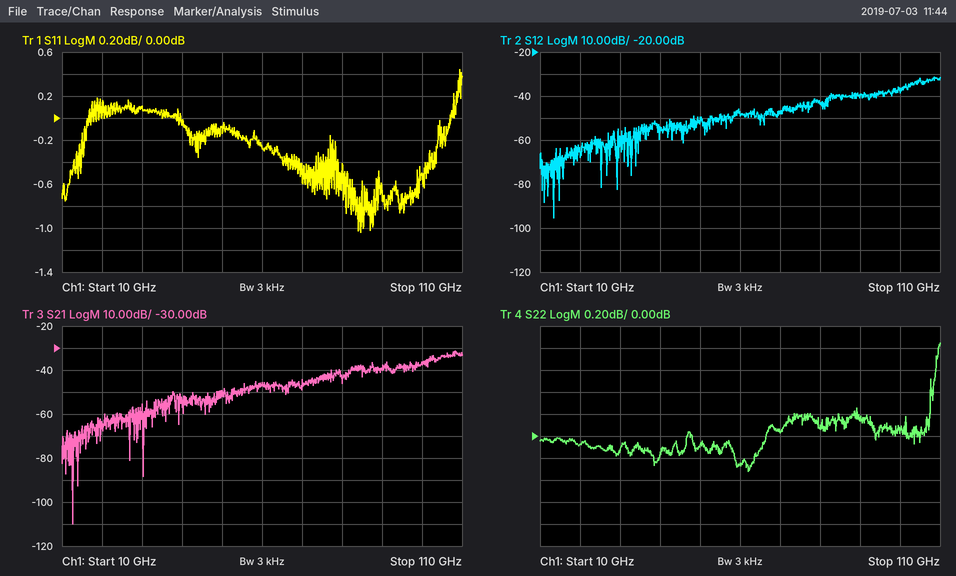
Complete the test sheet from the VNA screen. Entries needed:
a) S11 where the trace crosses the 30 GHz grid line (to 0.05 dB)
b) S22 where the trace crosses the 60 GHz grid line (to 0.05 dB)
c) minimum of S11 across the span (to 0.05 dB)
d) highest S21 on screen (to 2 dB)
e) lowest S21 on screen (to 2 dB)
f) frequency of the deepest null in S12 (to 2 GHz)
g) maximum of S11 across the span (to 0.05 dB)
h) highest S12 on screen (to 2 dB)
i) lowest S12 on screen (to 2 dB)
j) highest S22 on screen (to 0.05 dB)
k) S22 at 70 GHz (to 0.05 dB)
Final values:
0.10 dB
-0.25 dB
-1.05 dB
-32 dB
-110 dB
14 GHz
0.45 dB
-32 dB
-96 dB
0.85 dB
0.05 dB
